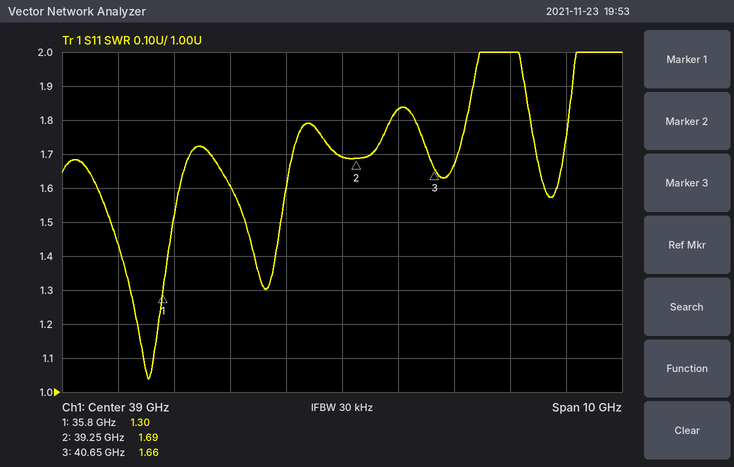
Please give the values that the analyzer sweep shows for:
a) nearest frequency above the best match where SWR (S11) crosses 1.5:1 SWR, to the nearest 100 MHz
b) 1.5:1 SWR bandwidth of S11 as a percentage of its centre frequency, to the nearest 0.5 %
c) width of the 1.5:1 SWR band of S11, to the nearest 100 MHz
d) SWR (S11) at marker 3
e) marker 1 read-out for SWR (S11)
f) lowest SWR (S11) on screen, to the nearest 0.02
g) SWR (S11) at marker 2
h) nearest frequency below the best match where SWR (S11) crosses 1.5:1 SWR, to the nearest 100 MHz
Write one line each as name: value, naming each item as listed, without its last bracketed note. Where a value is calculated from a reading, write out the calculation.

nearest frequency above the best match where SWR (S11) crosses 1.5:1 SWR, to the nearest 100 MHz: 36.0 GHz
1.5:1 SWR bandwidth of S11 as a percentage of its centre frequency, to the nearest 0.5 %: 1.1 GHz / 35.45 GHz ≈ 3.10 %, so 3.0 % to the nearest 0.5 %
width of the 1.5:1 SWR band of S11, to the nearest 100 MHz: 36.0 GHz − 34.9 GHz = 1.1 GHz
SWR (S11) at marker 3: 1.66
marker 1 read-out for SWR: 1.30
lowest SWR (S11) on screen, to the nearest 0.02: 1.04
SWR (S11) at marker 2: 1.69
nearest frequency below the best match where SWR (S11) crosses 1.5:1 SWR, to the nearest 100 MHz: 34.9 GHz
